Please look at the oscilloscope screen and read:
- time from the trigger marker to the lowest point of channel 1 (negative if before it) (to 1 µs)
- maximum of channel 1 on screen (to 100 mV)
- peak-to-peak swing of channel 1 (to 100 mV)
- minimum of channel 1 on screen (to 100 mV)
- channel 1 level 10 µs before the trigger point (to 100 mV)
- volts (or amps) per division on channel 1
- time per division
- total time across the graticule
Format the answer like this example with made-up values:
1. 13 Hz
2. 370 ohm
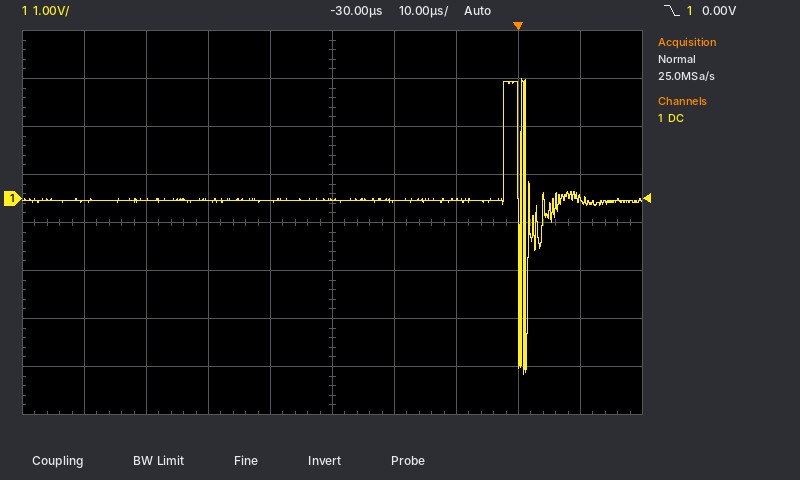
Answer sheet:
1. +1 µs
2. 2.5 V
3. 6.2 V
4. -3.7 V
5. 0.0 V
6. 1 V
7. 10 µs
8. 100 µs
